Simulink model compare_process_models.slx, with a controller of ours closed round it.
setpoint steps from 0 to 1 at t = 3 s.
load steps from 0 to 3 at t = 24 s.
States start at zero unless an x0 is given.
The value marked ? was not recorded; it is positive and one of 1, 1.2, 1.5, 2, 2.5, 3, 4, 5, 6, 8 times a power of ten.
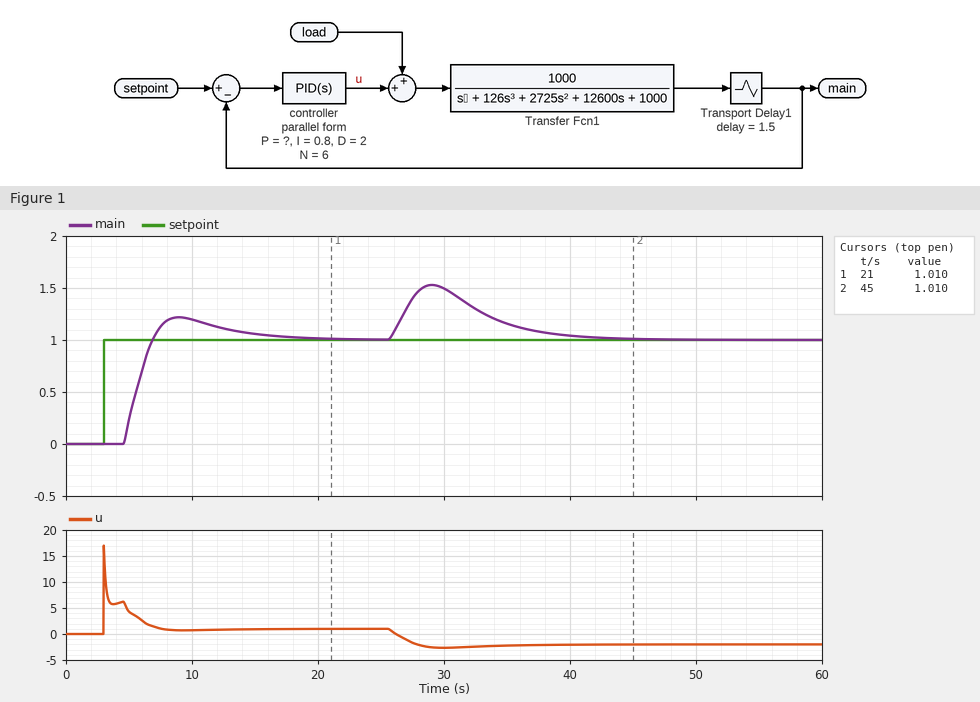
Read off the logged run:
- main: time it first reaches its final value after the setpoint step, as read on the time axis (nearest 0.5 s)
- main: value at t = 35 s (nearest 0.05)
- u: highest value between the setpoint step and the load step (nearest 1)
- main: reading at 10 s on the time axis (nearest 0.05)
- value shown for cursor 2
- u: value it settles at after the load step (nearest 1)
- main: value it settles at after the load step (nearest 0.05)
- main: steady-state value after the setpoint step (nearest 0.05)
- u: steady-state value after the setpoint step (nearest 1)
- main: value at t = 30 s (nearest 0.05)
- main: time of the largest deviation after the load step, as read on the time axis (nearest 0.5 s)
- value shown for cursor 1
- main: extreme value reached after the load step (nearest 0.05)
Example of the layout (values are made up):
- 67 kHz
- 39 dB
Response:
- 7.0 s
- 1.15
- 17
- 1.20
- 1.010
- -2
- 1.00
- 1.00
- 1
- 1.50
- 29.0 s
- 1.010
- 1.55
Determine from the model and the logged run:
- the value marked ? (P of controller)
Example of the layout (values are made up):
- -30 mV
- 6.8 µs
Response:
- 5
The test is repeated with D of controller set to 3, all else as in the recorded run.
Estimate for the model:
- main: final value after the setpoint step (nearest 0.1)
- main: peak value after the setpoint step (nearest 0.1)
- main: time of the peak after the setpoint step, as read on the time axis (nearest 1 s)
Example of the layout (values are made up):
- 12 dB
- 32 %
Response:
- 1.0
- 1.1
- 9 s
